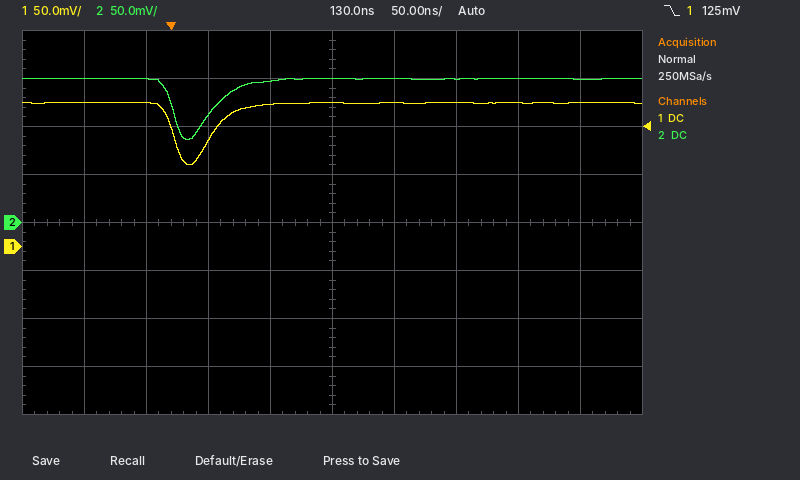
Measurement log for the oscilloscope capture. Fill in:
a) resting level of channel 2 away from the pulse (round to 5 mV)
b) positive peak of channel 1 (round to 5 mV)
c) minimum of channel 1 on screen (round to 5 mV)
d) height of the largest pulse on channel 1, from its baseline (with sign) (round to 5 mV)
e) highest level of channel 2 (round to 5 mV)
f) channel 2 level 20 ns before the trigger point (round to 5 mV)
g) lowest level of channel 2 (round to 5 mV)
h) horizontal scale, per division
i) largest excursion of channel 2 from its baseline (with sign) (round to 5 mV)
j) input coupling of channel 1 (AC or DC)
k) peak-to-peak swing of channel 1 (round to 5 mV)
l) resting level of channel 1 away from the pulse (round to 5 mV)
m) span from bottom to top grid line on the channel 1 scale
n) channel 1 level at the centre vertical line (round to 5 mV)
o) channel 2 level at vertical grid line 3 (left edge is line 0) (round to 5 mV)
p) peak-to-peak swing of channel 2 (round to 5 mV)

150 mV
150 mV
85 mV
-65 mV
150 mV
150 mV
85 mV
50 ns
-65 mV
DC
65 mV
150 mV
400 mV
150 mV
110 mV
65 mV
